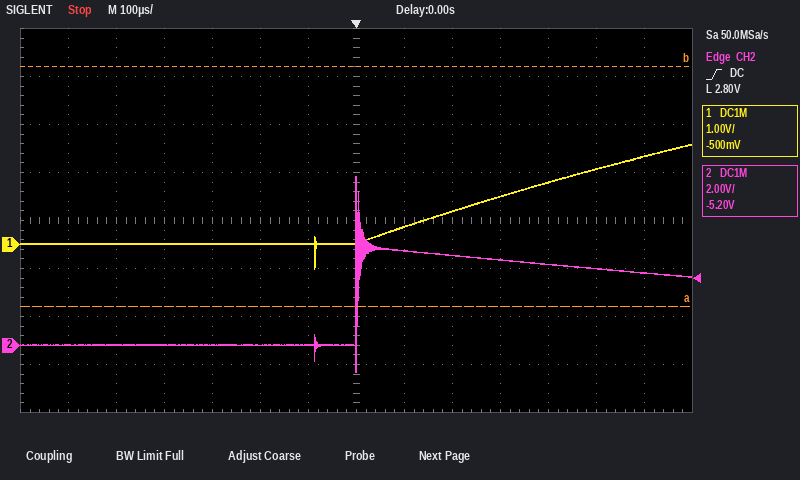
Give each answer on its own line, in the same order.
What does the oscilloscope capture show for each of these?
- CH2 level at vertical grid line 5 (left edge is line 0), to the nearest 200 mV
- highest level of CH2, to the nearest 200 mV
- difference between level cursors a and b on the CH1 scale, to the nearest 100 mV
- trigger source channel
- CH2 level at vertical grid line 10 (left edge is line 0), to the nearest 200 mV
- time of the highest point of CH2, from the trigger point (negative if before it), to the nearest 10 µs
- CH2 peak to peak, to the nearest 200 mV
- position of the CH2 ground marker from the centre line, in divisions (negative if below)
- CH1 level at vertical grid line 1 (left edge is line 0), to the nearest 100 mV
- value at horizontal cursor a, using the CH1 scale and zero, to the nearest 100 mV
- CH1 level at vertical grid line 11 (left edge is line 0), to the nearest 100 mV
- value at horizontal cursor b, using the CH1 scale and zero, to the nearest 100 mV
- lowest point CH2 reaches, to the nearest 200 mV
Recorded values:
0.0 V
7.0 V
5.0 V
CH2
3.6 V
0 µs
8.2 V
-2.6 div
0.0 V
-1.3 V
1.3 V
3.7 V
-1.2 V
